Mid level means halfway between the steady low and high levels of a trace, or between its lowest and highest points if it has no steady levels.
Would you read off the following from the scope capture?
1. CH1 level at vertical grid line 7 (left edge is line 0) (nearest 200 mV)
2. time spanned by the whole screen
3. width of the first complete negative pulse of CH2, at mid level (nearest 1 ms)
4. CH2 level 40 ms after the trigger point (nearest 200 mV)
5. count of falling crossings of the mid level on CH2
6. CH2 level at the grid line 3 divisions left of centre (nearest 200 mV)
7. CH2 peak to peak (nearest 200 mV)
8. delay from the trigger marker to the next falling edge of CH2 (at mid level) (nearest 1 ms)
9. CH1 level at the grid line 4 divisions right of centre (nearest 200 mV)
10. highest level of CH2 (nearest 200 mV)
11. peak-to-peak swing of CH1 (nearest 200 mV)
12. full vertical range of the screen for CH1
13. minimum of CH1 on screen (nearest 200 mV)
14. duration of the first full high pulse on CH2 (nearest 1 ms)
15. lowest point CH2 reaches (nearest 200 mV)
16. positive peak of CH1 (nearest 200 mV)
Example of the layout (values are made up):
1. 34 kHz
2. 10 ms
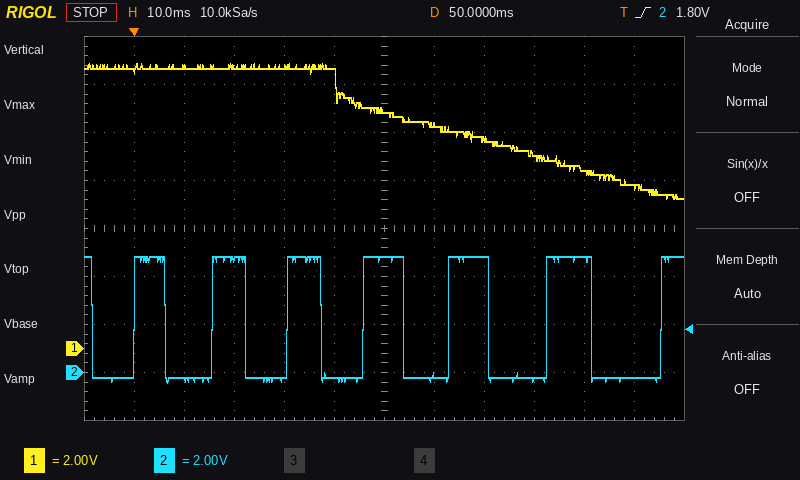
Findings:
1. 9.4 V
2. 120 ms
3. 8 ms
4. -200 mV
5. 7
6. 4.8 V
7. 5.2 V
8. 6 ms
9. 7.4 V
10. 4.8 V
11. 5.6 V
12. 16 V
13. 6.2 V
14. 6 ms
15. -400 mV
16. 11.8 V
